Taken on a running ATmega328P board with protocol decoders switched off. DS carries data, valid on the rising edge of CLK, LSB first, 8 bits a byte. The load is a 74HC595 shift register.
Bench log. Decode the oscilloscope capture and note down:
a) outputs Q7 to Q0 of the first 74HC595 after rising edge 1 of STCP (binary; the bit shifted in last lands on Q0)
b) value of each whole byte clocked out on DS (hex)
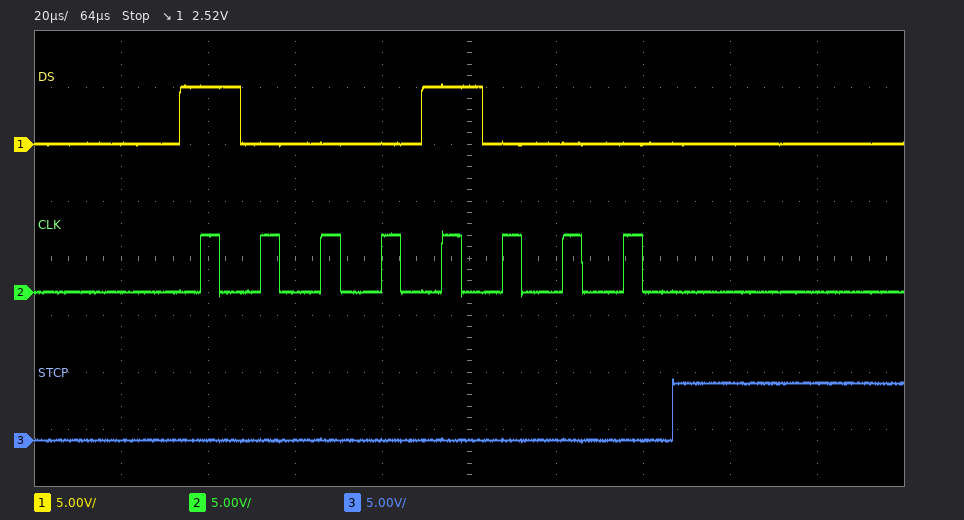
10001000
11
